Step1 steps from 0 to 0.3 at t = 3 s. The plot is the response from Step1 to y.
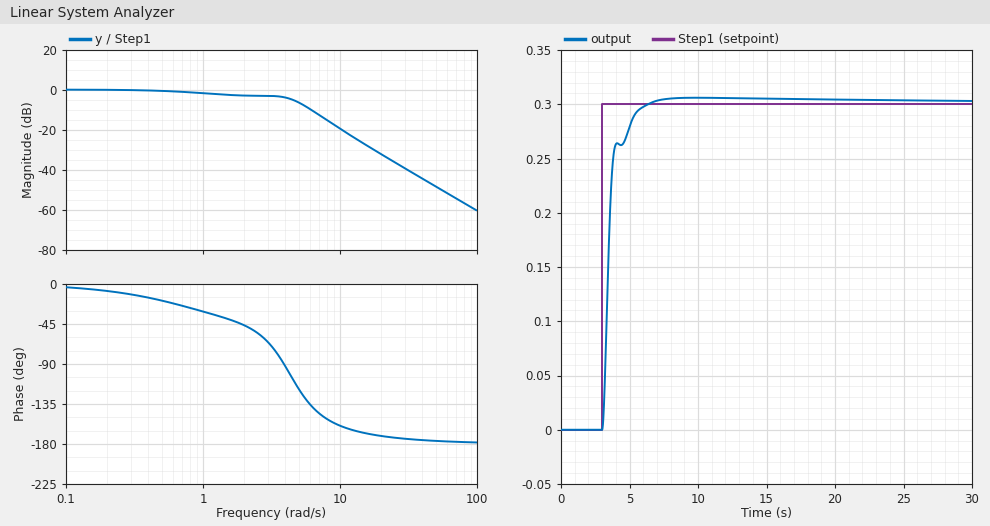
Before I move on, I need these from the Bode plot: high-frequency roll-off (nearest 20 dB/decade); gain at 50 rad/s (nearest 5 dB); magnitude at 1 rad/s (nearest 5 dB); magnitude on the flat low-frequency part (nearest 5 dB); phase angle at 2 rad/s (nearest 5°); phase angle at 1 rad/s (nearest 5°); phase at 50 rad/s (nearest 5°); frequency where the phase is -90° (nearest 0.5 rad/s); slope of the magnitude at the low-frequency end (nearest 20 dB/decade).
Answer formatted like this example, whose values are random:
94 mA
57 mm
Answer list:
-40 dB/decade
-50 dB
0 dB
0 dB
-45°
-30°
-175°
4.0 rad/s
0 dB/decade
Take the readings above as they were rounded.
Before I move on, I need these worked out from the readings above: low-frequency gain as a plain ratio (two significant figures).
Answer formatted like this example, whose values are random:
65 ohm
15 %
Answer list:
1.0
